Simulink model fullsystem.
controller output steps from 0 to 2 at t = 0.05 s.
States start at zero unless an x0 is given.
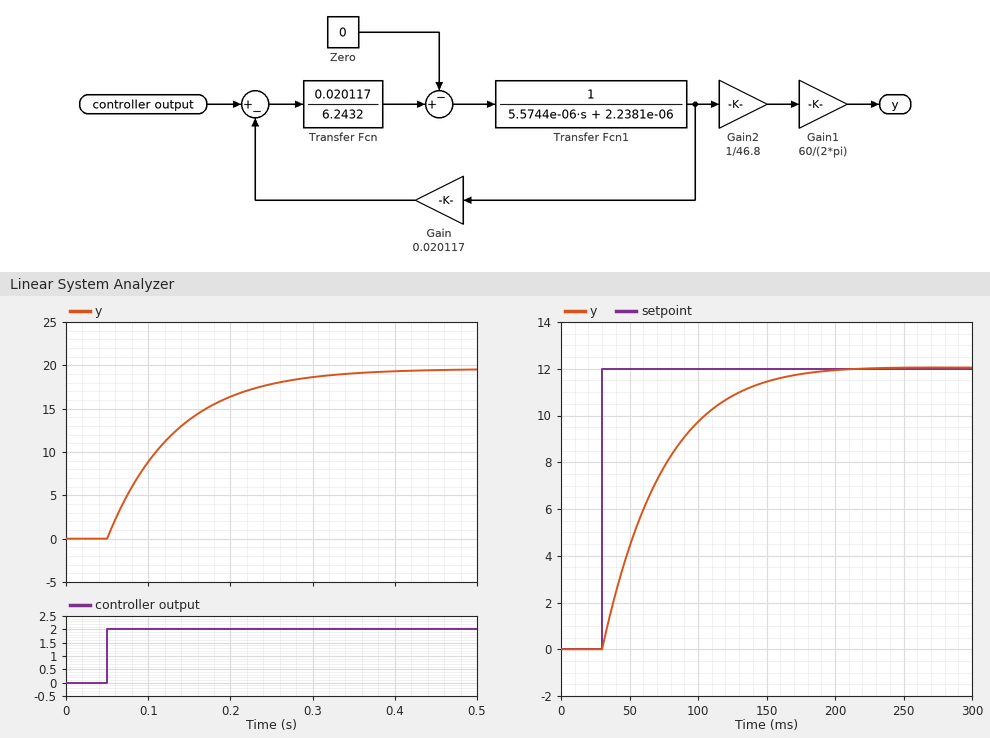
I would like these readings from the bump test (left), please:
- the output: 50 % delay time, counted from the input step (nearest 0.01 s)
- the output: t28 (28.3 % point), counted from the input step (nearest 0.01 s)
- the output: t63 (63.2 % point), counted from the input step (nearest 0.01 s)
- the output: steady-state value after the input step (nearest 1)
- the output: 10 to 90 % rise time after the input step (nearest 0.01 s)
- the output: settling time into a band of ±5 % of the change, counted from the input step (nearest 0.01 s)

0.06 s
0.03 s
0.08 s
20
0.18 s
0.25 s
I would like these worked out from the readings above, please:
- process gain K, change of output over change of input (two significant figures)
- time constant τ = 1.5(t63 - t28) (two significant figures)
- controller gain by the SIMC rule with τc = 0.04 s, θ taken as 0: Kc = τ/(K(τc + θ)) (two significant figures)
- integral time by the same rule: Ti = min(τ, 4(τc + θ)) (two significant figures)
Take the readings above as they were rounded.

10
0.075 s
0.19
0.075 s
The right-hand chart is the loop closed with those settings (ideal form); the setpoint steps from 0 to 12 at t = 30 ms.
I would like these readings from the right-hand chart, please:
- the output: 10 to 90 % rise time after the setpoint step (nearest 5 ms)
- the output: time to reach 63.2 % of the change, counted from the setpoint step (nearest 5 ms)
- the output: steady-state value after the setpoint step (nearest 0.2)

90 ms
45 ms
12.0
